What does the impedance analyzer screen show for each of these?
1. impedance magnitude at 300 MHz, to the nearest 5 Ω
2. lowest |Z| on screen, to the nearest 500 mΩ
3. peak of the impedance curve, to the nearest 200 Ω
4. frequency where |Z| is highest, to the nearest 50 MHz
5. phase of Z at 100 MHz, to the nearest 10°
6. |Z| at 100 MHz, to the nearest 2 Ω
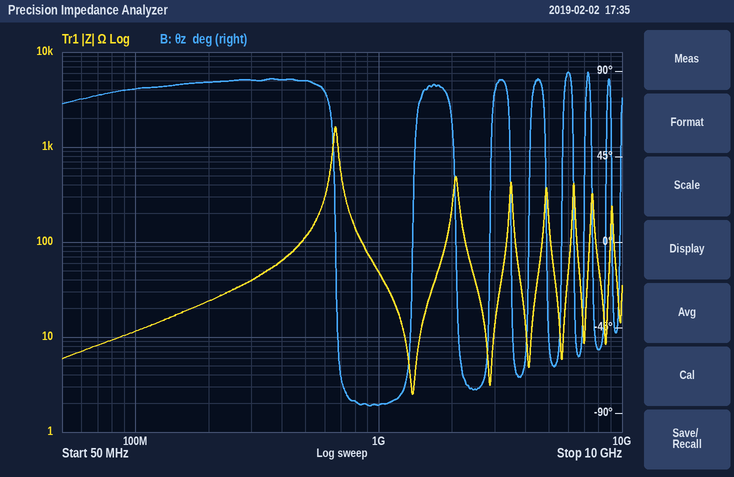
40 Ω
2.5 Ω
1.6 kΩ
650 MHz
80°
12 Ω
